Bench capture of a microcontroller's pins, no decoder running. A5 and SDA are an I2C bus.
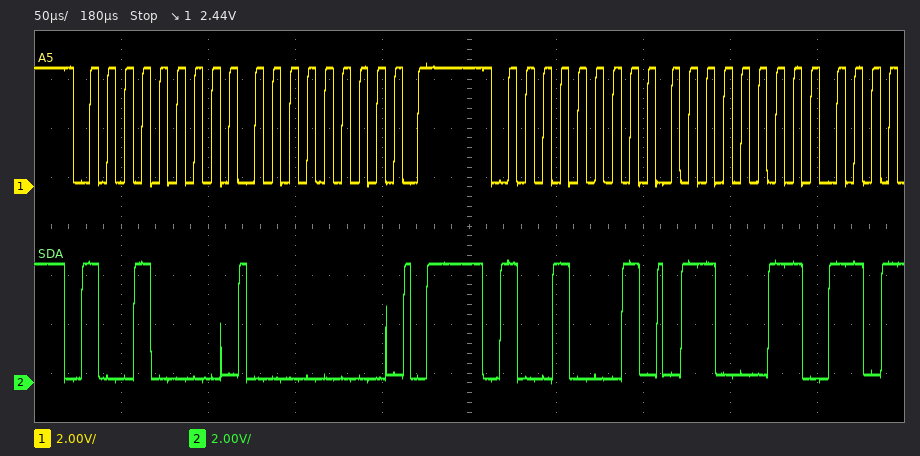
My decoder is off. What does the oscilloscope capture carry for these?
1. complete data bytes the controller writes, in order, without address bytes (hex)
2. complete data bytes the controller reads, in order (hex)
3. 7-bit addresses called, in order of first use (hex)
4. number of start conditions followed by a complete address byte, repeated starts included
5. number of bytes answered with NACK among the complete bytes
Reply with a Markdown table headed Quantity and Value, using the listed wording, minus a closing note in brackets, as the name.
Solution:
| Quantity | Value |
|---|---|
| complete data bytes the controller writes, in order, without address bytes | 00 |
| complete data bytes the controller reads, in order | 63 |
| 7-bit addresses called, in order of first use | 0x48 |
| number of start conditions followed by a complete address byte, repeated starts included | 2 |
| number of bytes answered with NACK among the complete bytes | 0 |
